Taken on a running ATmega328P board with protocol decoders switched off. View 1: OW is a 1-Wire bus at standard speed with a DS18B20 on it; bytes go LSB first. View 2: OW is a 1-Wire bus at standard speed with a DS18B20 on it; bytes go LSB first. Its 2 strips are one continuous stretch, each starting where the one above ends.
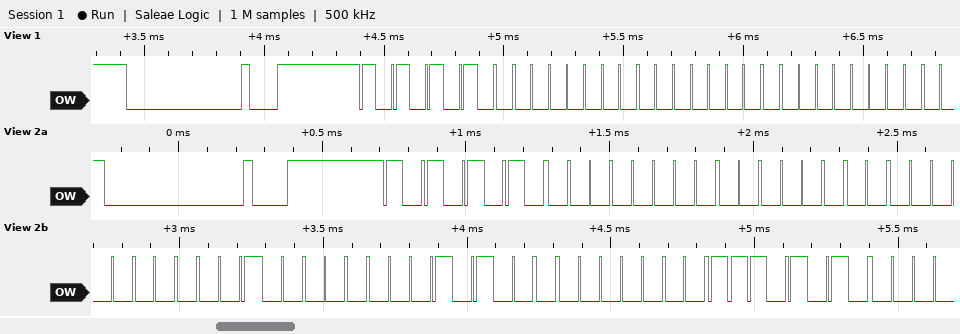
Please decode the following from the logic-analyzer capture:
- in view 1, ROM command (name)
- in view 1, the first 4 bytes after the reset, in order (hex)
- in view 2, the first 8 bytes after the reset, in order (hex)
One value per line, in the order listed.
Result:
Match ROM
55 00 00 00
55 00 00 00 04 28 00 57
